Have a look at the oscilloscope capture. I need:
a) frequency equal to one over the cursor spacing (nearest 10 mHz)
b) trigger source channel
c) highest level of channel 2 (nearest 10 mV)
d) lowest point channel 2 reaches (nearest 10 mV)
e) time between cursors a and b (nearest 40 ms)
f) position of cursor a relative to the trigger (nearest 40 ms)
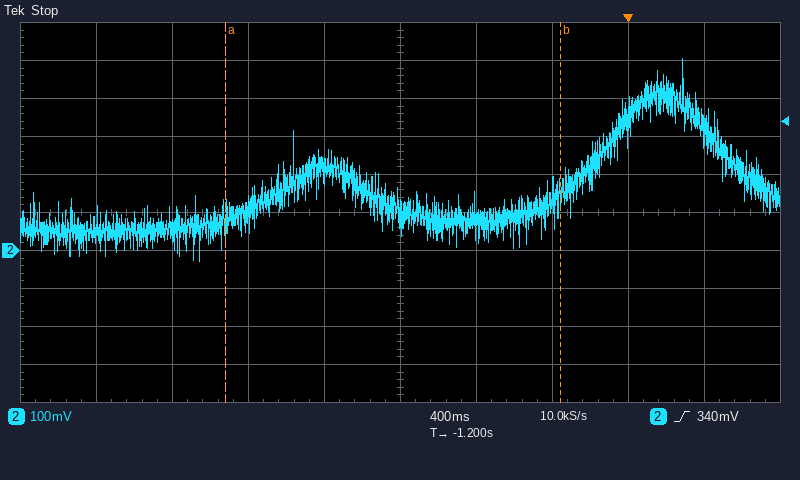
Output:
570 mHz
channel 2
510 mV
-30 mV
1.76 s
-2.12 s
